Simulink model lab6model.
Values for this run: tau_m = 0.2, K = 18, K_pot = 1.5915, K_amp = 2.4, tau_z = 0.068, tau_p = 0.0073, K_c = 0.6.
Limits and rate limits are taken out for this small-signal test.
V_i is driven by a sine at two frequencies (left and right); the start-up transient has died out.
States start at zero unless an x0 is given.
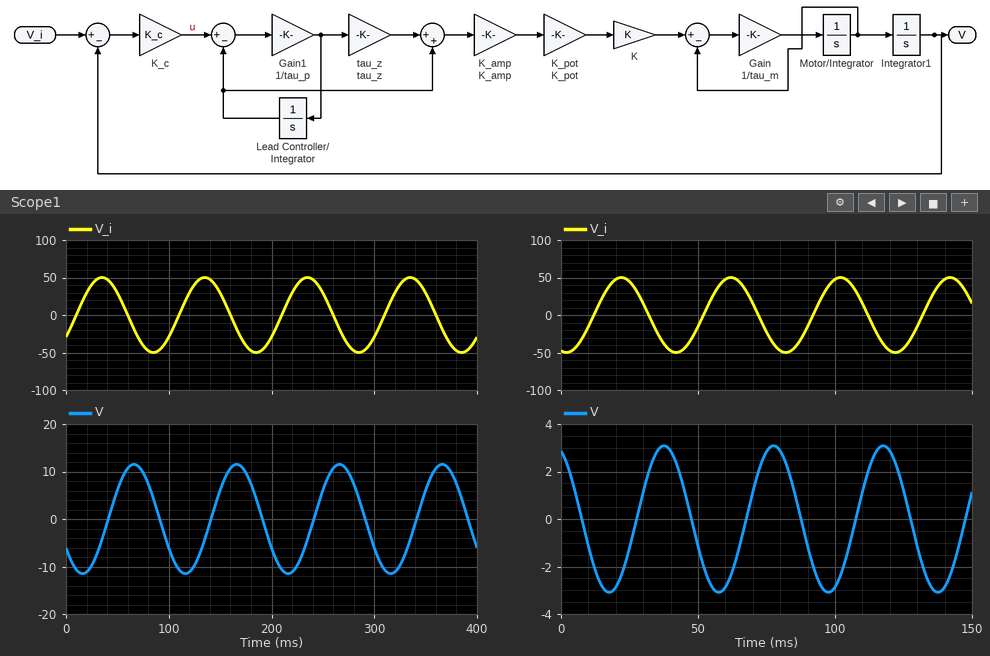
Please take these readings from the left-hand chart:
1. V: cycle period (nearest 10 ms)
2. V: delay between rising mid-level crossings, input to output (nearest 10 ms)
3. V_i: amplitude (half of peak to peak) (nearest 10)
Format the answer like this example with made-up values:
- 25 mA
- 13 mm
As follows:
- 100 ms
- 30 ms
- 50
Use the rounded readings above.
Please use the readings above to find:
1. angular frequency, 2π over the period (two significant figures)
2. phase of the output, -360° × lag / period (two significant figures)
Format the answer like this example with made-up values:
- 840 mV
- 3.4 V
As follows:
- 0.063 rad/ms
- -110°
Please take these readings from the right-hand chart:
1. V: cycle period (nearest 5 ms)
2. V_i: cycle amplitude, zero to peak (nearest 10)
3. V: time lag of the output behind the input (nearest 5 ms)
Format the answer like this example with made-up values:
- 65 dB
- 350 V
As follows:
- 40 ms
- 50
- 15 ms
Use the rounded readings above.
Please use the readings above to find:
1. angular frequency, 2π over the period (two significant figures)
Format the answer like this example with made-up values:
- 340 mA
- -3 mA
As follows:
- 0.16 rad/ms
